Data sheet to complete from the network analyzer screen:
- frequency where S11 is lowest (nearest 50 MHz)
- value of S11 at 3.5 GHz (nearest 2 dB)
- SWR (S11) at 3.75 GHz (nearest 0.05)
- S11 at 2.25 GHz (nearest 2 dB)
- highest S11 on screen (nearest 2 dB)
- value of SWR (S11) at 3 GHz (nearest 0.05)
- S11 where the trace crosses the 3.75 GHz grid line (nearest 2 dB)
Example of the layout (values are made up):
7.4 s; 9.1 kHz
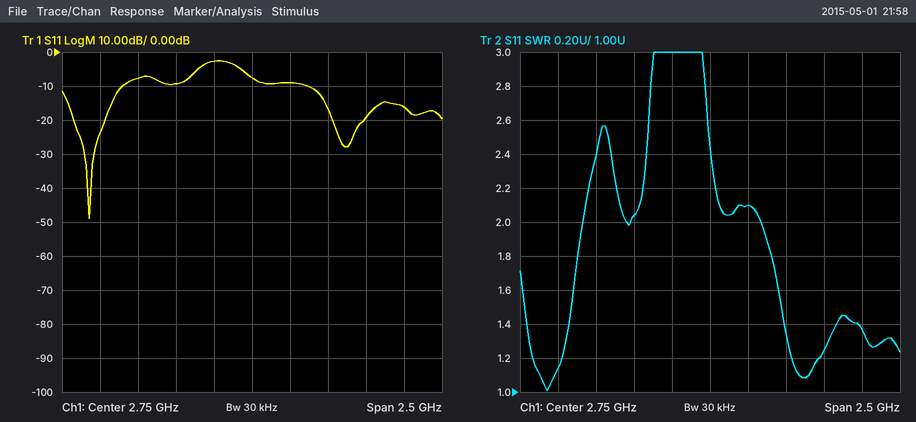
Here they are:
1.70 GHz; -20 dB; 1.35; -10 dB; -2 dB; 2.10; -16 dB
